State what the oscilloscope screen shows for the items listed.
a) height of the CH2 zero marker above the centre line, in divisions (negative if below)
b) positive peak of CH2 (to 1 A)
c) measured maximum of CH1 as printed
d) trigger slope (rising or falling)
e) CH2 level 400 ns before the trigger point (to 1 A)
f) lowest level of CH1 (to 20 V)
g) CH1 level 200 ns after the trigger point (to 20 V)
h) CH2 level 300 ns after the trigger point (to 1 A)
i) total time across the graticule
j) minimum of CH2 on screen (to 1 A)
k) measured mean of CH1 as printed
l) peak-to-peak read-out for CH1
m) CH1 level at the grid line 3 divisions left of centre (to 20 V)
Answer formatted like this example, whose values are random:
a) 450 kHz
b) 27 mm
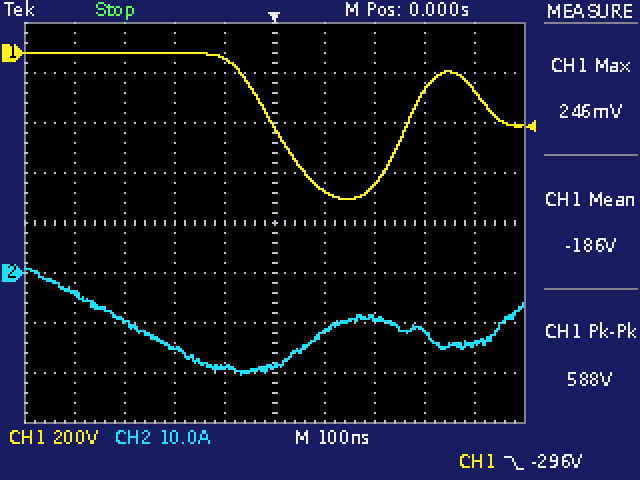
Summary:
a) -1.0 div
b) 1 A
c) 246 mV
d) falling
e) -4 A
f) -580 V
g) -520 V
h) -12 A
i) 1 µs
j) -20 A
k) -186 V
l) 588 V
m) 0 V
